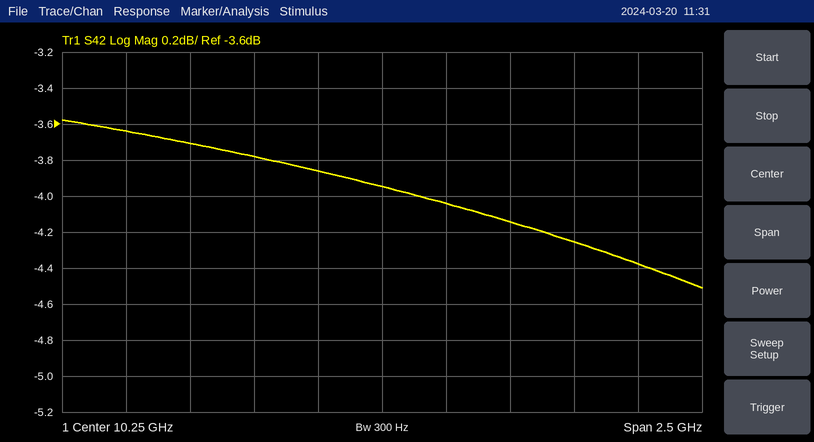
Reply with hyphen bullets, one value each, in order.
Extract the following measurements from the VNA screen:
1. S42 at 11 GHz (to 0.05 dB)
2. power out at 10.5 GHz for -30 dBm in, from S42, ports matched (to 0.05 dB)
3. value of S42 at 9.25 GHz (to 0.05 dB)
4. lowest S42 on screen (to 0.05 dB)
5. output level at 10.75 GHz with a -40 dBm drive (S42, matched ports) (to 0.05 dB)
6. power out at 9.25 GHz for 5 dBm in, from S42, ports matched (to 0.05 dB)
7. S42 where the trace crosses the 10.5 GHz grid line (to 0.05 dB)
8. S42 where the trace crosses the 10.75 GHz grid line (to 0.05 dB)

- -4.25 dB
- -34.05 dBm
- -3.65 dB
- -4.50 dB
- -44.15 dBm
- 1.35 dBm
- -4.05 dB
- -4.15 dB
